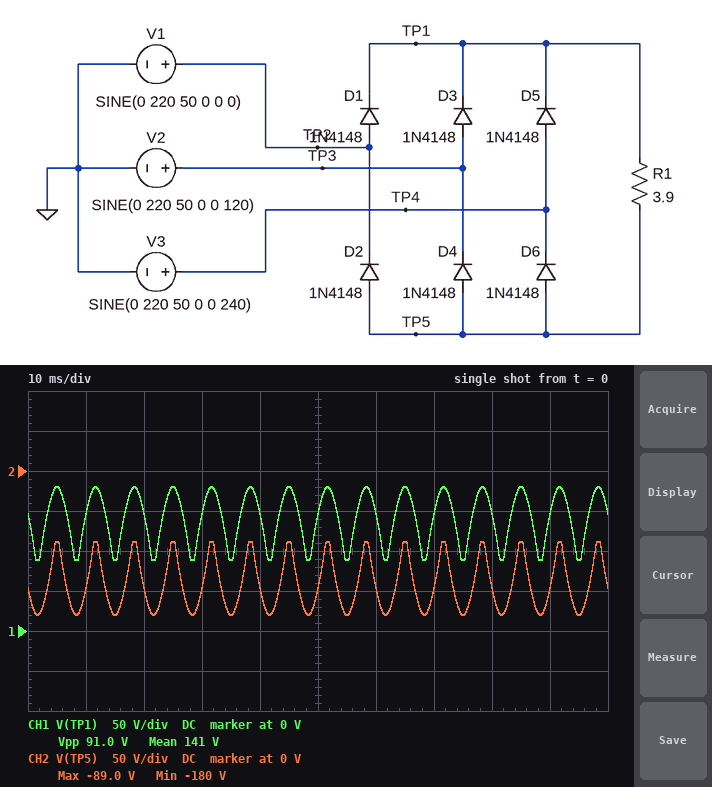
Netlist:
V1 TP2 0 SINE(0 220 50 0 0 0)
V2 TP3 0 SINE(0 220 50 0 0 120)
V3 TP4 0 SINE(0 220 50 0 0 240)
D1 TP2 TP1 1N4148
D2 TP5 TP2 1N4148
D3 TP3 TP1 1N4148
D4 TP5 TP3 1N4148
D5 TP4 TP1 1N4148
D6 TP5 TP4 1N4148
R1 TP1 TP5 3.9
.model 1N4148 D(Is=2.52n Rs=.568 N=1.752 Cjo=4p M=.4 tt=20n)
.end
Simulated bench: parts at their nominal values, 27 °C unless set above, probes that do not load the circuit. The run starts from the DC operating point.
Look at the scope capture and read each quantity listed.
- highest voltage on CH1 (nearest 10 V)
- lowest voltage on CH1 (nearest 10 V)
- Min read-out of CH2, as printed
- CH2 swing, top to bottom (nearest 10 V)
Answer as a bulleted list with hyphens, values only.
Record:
- 180 V
- 90 V
- -180 V
- 90 V
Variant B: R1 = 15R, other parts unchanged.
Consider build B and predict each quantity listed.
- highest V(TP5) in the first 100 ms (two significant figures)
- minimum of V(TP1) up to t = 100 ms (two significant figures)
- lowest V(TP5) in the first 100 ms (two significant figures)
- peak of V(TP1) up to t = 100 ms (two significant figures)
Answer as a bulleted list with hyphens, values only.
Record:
- -100 V
- 100 V
- -210 V
- 210 V
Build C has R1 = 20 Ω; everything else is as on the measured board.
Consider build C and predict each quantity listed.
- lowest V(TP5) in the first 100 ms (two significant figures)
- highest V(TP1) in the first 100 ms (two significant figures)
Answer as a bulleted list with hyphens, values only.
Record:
- -210 V
- 210 V
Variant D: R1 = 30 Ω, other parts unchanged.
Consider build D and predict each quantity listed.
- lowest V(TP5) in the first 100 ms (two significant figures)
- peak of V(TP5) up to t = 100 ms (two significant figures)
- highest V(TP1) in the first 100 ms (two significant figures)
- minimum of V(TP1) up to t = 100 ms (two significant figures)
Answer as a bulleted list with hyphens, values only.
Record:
- -210 V
- -110 V
- 210 V
- 110 V
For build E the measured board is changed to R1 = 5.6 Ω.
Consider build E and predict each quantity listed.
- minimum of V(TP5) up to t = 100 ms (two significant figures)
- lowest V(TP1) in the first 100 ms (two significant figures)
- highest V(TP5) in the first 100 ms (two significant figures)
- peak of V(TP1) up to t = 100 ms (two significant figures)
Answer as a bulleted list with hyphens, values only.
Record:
- -190 V
- 94 V
- -94 V
- 190 V
